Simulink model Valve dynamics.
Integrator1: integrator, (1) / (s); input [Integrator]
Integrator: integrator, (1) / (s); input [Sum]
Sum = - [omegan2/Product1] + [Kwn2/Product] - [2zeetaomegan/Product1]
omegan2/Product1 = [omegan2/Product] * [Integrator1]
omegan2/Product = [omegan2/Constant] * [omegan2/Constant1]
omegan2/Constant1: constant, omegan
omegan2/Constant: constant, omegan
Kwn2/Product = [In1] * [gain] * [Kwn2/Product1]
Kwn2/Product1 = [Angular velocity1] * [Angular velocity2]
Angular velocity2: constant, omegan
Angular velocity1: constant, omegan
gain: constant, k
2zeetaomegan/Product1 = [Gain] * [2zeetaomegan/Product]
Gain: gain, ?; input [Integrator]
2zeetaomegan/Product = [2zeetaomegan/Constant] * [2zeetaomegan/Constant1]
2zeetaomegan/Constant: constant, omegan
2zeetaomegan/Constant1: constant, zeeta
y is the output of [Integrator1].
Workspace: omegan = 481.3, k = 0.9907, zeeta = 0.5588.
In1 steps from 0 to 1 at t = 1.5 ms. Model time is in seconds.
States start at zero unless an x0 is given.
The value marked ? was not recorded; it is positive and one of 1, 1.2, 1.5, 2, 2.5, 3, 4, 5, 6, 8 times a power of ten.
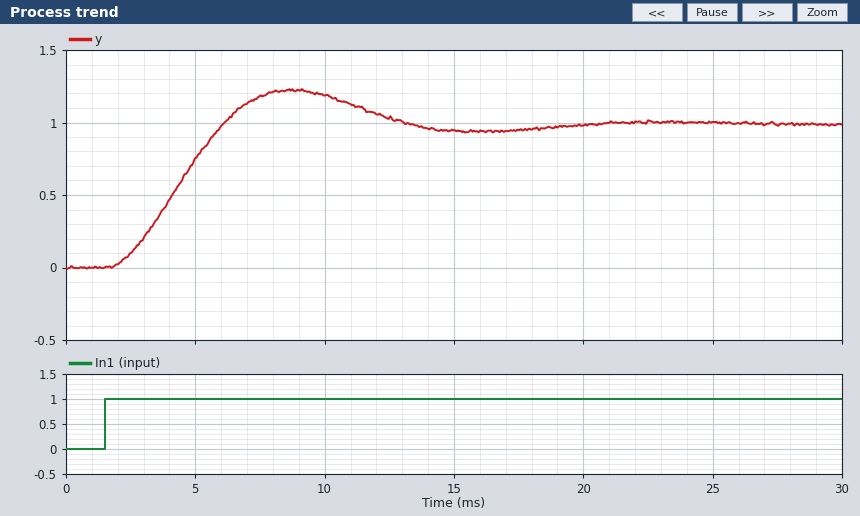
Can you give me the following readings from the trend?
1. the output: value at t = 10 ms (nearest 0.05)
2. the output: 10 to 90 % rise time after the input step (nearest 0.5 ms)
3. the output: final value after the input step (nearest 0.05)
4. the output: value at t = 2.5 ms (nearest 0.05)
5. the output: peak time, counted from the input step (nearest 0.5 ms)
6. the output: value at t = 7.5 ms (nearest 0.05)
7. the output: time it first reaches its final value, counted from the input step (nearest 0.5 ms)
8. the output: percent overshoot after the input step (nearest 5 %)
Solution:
1.20
3.0 ms
1.00
0.10
7.0 ms
1.20
4.5 ms
25 %
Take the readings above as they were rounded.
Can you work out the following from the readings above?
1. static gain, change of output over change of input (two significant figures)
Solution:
1.0
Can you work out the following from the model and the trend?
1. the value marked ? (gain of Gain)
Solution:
1.5
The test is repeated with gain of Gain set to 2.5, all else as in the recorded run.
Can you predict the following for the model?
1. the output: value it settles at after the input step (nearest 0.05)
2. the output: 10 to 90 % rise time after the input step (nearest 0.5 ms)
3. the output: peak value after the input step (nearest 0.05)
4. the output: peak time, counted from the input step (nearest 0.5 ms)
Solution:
1.00
4.5 ms
1.05
9.0 ms
